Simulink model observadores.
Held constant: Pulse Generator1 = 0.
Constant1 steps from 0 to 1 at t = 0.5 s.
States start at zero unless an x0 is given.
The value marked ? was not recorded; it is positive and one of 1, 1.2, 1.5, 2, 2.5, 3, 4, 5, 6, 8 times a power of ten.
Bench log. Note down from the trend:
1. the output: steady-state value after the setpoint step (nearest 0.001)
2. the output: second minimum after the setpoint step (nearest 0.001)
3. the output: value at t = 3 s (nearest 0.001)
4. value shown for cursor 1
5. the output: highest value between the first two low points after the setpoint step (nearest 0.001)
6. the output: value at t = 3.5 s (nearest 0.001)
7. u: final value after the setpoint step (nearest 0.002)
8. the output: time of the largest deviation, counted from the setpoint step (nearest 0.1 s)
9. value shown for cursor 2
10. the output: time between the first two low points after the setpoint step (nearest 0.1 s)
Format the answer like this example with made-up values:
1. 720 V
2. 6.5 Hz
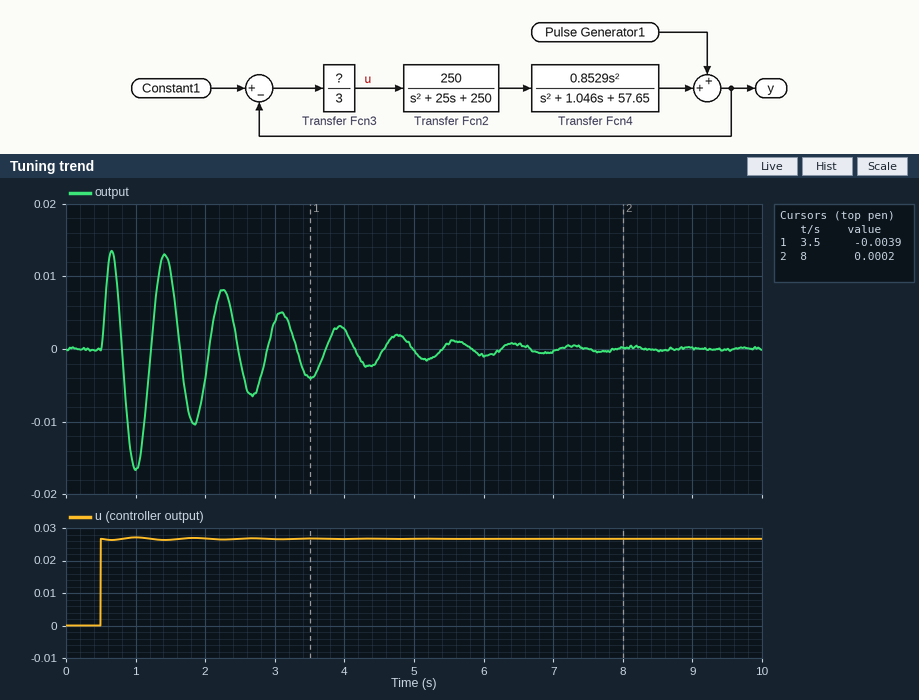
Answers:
1. 0.000
2. -0.010
3. 0.004
4. -0.0039
5. 0.013
6. -0.004
7. 0.026
8. 0.5 s
9. 0.0002
10. 0.8 s
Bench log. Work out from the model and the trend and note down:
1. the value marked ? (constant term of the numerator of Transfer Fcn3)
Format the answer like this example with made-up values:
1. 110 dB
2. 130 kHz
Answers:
1. 0.08
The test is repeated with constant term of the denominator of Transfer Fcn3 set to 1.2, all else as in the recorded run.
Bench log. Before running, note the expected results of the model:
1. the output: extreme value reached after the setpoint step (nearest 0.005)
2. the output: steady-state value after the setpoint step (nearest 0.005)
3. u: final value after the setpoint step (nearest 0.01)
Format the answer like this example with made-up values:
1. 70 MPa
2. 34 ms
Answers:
1. -0.040
2. 0.000
3. 0.07
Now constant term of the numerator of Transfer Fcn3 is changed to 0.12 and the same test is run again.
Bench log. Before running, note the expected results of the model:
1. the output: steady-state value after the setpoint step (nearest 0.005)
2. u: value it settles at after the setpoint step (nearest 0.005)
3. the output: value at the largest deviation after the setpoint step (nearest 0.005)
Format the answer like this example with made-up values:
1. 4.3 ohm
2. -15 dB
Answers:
1. 0.000
2. 0.040
3. -0.025
